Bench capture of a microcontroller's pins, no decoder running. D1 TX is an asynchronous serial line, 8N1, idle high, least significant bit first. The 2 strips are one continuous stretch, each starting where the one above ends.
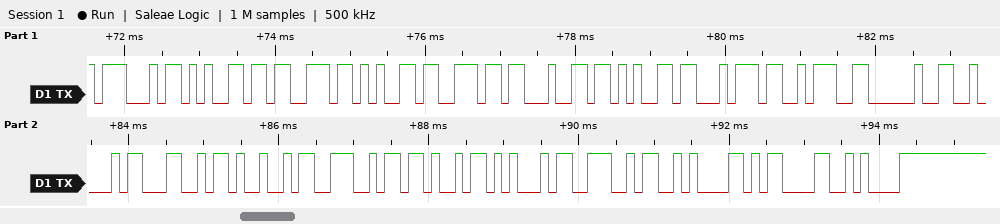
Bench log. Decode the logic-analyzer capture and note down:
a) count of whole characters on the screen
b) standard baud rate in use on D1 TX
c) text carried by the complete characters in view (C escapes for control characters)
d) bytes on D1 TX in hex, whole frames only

20
9600 baud
"Gesendet: BLINKEN\n\r\n"
47 65 73 65 6E 64 65 74 3A 20 42 4C 49 4E 4B 45 4E 0A 0D 0A
